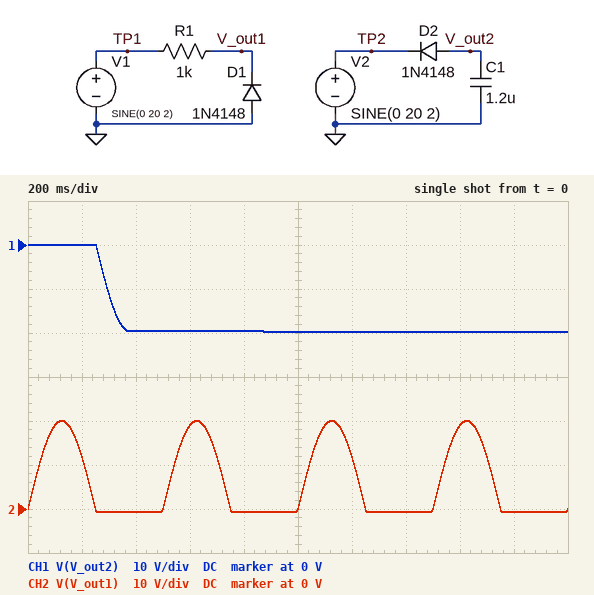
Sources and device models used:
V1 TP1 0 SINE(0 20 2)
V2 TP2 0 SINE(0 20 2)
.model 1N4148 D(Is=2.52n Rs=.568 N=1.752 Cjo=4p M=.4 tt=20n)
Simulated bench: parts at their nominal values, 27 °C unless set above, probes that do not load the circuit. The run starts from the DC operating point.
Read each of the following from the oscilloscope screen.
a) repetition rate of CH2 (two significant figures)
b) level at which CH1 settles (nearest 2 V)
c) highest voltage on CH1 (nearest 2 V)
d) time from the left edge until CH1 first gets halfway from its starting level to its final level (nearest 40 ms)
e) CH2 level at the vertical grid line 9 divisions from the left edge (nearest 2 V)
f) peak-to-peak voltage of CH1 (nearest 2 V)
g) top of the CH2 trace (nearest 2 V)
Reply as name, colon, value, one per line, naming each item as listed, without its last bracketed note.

repetition rate of CH2: 2.0 Hz
level at which CH1 settles: -20 V
highest voltage on CH1: 0 V
time from the left edge until CH1 first gets halfway from its starting level to its final level: 280 ms
CH2 level at the vertical grid line 9 divisions from the left edge: 0 V
peak-to-peak voltage of CH1: 20 V
top of the CH2 trace: 20 V
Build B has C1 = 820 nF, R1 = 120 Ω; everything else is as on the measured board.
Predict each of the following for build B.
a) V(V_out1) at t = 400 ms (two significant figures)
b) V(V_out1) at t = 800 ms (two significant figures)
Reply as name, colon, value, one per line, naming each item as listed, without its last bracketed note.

V(V_out1) at t = 400 ms: -900 mV
V(V_out1) at t = 800 ms: -840 mV
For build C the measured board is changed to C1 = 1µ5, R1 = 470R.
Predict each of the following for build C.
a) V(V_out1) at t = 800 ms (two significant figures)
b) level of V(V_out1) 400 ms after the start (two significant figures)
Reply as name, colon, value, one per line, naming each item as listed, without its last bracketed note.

V(V_out1) at t = 800 ms: -740 mV
level of V(V_out1) 400 ms after the start: -770 mV
